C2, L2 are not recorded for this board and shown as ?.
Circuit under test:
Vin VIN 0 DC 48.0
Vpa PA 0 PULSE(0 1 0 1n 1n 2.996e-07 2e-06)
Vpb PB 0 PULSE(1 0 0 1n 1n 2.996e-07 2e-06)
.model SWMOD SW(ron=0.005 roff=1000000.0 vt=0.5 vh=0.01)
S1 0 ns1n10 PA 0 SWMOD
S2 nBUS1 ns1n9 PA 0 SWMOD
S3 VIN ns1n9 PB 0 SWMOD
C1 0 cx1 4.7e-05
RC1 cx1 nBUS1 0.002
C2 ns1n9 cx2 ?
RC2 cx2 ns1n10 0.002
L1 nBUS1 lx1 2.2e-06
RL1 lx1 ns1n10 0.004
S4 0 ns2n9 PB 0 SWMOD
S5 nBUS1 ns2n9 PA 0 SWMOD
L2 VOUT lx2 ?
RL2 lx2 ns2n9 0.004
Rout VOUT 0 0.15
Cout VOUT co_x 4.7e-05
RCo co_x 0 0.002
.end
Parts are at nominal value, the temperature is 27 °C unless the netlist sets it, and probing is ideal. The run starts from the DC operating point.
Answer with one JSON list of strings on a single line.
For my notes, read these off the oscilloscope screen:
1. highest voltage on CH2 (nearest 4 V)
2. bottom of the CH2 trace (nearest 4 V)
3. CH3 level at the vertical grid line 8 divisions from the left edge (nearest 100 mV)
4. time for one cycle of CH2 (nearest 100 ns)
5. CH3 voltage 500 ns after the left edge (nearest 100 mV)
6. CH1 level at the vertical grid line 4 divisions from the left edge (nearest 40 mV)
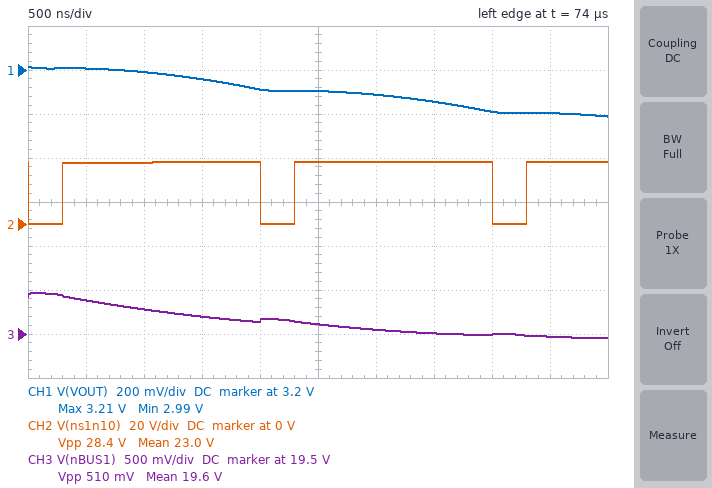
["28 V", "0 V", "19.5 V", "2.0 µs", "19.9 V", "3.12 V"]
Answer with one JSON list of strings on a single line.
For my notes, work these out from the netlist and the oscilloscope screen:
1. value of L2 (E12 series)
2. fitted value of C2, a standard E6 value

["1 µH", "68 µF"]
